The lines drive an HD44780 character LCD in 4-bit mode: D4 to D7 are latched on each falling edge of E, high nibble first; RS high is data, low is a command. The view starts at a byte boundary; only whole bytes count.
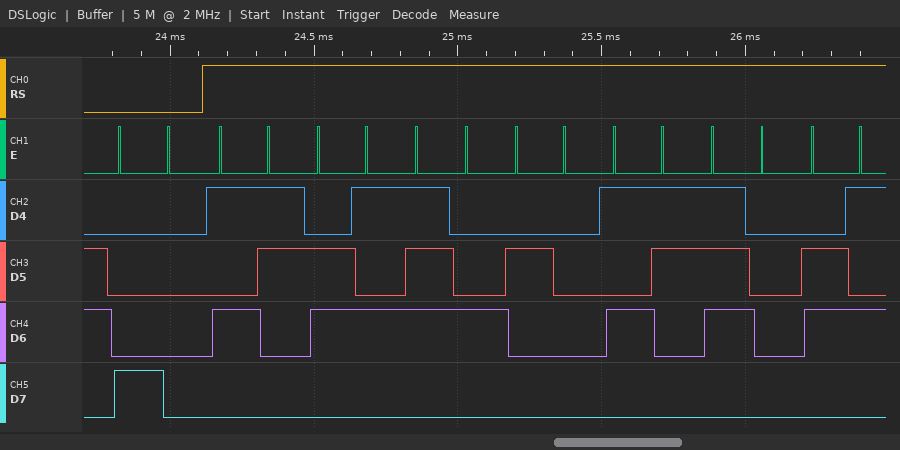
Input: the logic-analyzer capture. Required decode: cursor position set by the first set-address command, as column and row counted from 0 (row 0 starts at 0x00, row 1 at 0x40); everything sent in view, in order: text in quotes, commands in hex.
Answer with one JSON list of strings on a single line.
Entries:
["column 0, row 0", "0x80 \"Set Spe\""]
